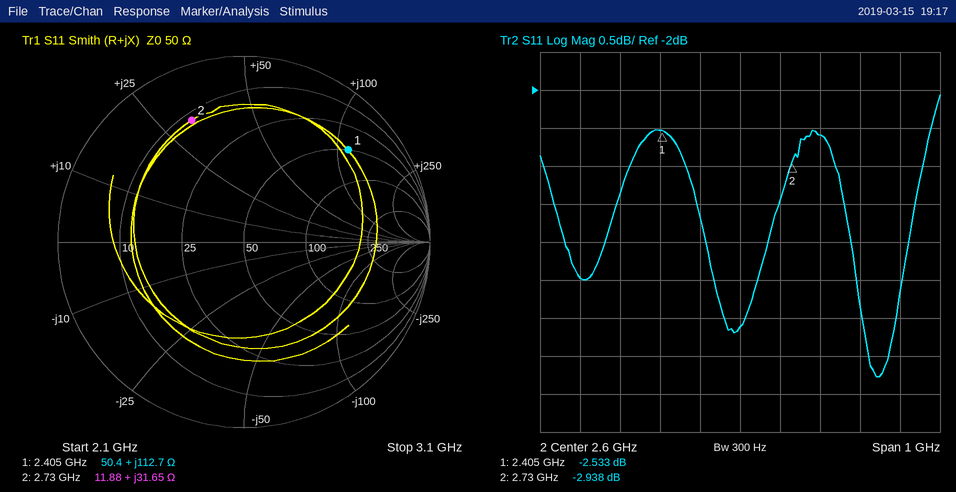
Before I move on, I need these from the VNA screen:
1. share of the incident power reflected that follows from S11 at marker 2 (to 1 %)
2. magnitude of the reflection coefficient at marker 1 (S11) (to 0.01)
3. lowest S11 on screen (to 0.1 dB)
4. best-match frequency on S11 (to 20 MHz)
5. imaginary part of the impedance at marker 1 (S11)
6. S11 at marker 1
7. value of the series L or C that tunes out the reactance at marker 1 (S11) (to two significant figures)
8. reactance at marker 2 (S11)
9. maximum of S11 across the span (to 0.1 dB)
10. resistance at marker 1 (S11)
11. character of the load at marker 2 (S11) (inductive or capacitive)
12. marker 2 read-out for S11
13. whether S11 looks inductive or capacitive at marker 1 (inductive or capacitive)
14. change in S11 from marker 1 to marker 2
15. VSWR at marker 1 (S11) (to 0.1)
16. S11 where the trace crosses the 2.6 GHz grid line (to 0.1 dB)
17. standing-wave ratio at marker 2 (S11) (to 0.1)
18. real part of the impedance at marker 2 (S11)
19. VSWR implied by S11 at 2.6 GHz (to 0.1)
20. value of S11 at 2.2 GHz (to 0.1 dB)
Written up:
51 %
0.75
-5.8 dB
2.94 GHz
+112.7 Ω
-2.533 dB
590 fF
+31.65 Ω
-2.1 dB
50.4 Ω
inductive
-2.938 dB
inductive
-0.405 dB
6.9
-5.1 dB
6.0
11.88 Ω
3.5
-4.5 dB
